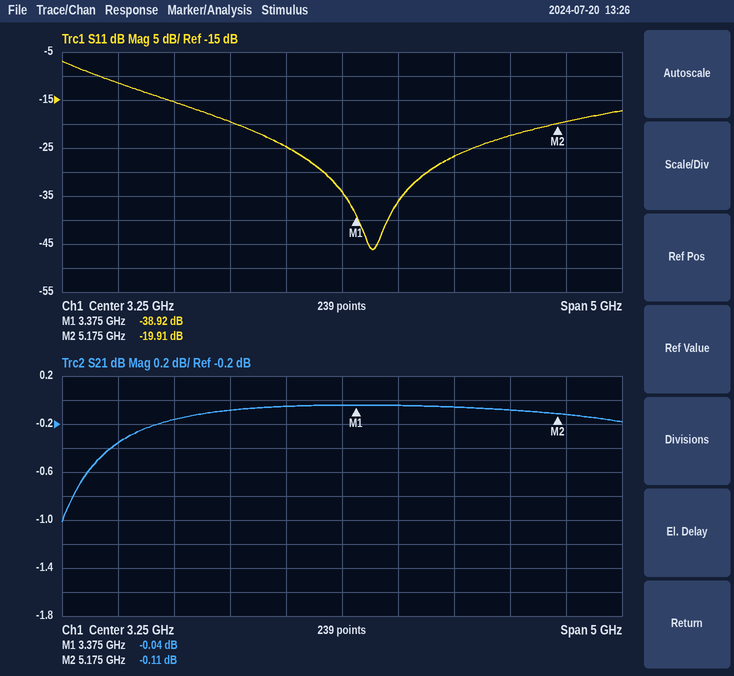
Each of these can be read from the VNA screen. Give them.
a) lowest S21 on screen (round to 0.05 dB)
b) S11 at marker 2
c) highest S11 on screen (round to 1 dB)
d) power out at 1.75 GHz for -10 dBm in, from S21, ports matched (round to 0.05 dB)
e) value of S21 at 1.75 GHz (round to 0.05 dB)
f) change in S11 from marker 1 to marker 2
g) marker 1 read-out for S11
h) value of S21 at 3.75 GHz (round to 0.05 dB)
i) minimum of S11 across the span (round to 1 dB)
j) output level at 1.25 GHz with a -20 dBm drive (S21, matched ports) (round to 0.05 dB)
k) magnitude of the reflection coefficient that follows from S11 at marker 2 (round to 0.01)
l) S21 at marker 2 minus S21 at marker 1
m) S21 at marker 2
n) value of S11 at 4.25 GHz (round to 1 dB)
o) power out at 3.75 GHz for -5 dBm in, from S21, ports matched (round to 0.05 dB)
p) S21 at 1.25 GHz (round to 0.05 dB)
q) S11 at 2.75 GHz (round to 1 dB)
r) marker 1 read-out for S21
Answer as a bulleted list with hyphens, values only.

- -1.00 dB
- -19.91 dB
- -7 dB
- -10.15 dBm
- -0.15 dB
- 19.01 dB
- -38.92 dB
- -0.05 dB
- -46 dB
- -20.35 dBm
- 0.10
- -0.07 dB
- -0.11 dB
- -27 dB
- -5.05 dBm
- -0.35 dB
- -25 dB
- -0.04 dB
